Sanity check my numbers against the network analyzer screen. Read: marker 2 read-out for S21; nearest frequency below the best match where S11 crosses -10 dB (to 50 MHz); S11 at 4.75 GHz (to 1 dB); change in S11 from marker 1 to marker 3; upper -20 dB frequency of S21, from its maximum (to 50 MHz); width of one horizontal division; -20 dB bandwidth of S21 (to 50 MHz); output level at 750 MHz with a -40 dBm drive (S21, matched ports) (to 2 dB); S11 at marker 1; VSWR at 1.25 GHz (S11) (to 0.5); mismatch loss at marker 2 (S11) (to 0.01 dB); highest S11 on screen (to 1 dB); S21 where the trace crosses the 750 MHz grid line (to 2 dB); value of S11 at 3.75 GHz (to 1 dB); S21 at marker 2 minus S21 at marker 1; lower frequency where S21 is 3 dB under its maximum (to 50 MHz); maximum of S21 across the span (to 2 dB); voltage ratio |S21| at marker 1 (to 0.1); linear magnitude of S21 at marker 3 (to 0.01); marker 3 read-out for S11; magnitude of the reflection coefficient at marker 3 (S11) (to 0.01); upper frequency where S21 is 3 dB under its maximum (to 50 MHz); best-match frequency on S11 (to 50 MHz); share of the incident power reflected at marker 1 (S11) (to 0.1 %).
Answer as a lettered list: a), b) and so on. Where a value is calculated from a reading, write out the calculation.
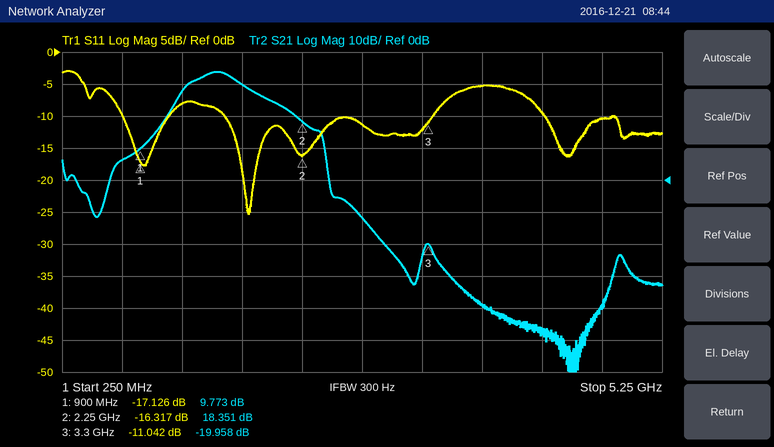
a) 18.351 dB
b) 1.60 GHz
c) -10 dB
d) -11.042 − (-17.126) = 6.084 dB
e) 2.40 GHz
f) 500 MHz
g) 2.40 GHz − 1.00 GHz = 1.40 GHz
h) -40 dBm + (6 dB) = -34 dBm
i) -17.126 dB
j) |Γ| = 10^(-8/20) = 0.3981; VSWR = (1 + 0.3981)/(1 − 0.3981) ≈ 2.32, so 2.5 to the nearest 0.5
k) −10 log10(1 − 10^(-16.317/10)) ≈ 0.10 dB
l) -3 dB
m) 6 dB
n) -5 dB
o) 18.351 − (9.773) = 8.578 dB
p) 1.35 GHz
q) 34 dB
r) 10^(9.773/20) ≈ 3.1
s) 10^(-19.958/20) ≈ 0.10
t) -11.042 dB
u) 10^(-11.042/20) ≈ 0.28
v) 1.70 GHz
w) 1.80 GHz
x) 10^(-17.126/10) ≈ 1.9 %
